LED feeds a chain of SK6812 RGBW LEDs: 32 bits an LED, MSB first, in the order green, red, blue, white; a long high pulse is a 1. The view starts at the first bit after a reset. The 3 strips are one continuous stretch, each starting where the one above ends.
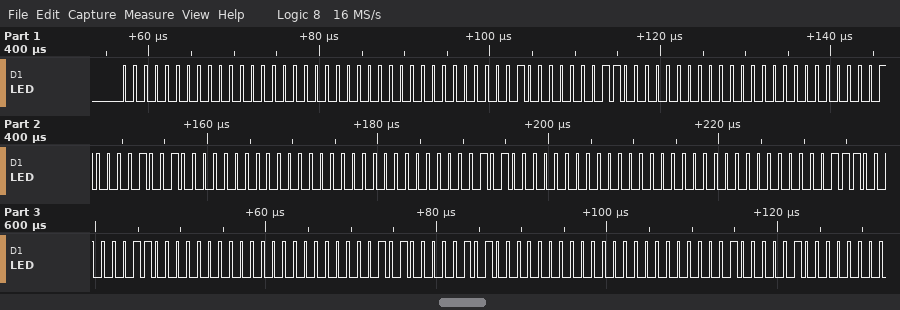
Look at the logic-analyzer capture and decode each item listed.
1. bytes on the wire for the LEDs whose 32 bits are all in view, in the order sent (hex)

00 00 00 00 04 06 00 00 01 09 00 00 00 0A 00 00 00 07 03 00 00 05 05 00
